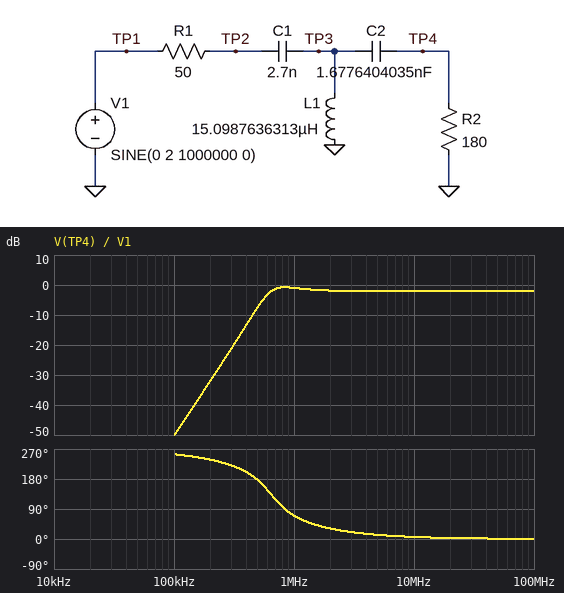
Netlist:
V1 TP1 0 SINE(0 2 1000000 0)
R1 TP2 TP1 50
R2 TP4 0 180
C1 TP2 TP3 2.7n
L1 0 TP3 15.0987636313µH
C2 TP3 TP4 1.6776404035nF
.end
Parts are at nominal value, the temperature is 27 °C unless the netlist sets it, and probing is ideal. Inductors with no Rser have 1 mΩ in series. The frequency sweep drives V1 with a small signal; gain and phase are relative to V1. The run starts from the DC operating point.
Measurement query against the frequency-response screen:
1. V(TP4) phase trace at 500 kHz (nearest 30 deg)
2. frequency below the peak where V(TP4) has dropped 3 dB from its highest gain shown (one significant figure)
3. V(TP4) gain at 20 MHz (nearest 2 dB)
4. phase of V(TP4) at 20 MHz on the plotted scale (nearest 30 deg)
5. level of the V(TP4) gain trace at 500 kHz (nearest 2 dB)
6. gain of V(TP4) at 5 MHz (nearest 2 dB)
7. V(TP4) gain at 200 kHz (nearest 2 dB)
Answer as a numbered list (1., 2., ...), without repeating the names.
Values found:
1. 180 deg
2. 600 kHz
3. -2 dB
4. 0 deg
5. -8 dB
6. -2 dB
7. -32 dB
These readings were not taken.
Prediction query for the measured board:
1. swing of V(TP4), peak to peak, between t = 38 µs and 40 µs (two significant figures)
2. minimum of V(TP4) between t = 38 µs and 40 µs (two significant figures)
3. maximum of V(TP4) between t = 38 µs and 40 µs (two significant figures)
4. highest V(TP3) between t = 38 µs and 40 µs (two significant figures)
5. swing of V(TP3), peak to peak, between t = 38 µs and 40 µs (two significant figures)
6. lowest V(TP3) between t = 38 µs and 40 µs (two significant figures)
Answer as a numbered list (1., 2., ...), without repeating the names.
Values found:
1. 3.6 V
2. -1.8 V
3. 1.8 V
4. 2.0 V
5. 4.0 V
6. -2.0 V
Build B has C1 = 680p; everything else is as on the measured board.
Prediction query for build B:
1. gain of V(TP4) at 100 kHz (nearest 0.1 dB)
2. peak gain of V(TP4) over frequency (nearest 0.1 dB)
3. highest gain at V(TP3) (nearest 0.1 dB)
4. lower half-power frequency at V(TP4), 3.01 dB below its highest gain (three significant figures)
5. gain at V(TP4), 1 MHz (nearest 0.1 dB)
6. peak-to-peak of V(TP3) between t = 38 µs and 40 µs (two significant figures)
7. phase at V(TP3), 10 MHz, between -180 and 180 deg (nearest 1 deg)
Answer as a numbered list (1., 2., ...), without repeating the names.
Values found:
1. -62.3 dB
2. -1.3 dB
3. -0.9 dB
4. 1.05 MHz
5. -5.1 dB
6. 2.5 V
7. 8 deg
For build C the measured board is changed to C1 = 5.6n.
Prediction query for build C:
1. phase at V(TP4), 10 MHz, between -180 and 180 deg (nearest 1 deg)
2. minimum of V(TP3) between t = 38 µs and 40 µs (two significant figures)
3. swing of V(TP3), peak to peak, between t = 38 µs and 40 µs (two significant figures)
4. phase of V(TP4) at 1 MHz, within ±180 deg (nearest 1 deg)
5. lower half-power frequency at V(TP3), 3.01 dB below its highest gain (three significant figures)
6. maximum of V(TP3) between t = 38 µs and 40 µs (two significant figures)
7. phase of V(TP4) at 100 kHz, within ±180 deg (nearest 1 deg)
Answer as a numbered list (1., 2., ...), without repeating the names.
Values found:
1. 5 deg
2. -1.8 V
3. 3.6 V
4. 56 deg
5. 406 kHz
6. 1.8 V
7. -111 deg
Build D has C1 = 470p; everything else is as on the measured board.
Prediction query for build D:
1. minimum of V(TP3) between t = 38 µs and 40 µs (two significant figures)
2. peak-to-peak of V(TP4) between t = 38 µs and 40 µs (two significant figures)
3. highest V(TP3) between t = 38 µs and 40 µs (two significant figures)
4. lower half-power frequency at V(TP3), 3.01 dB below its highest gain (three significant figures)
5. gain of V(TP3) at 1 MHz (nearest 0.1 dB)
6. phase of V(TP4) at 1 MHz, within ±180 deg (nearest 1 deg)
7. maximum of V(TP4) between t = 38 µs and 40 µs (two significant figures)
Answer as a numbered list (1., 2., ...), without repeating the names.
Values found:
1. -810 mV
2. 1.4 V
3. 810 mV
4. 1.23 MHz
5. -7.8 dB
6. 158 deg
7. 720 mV
